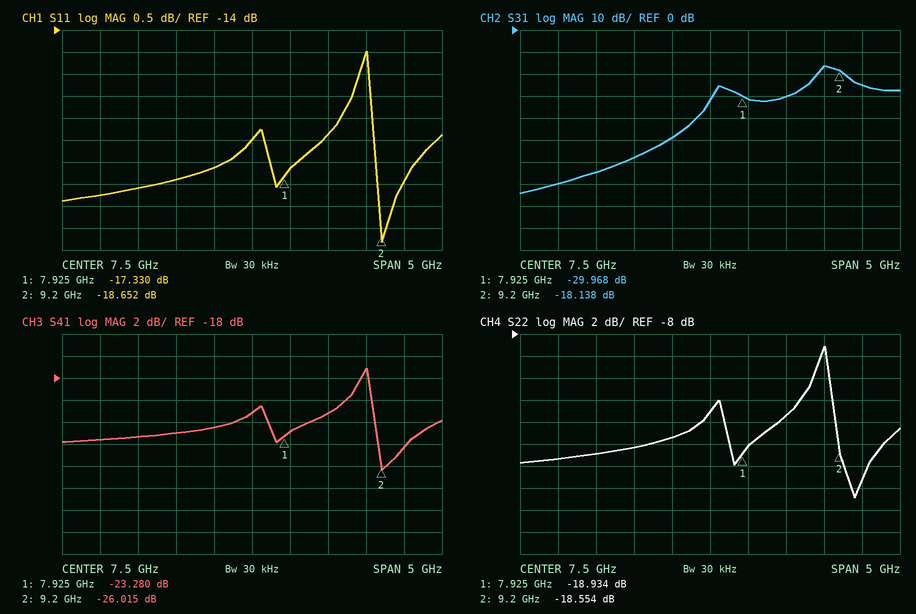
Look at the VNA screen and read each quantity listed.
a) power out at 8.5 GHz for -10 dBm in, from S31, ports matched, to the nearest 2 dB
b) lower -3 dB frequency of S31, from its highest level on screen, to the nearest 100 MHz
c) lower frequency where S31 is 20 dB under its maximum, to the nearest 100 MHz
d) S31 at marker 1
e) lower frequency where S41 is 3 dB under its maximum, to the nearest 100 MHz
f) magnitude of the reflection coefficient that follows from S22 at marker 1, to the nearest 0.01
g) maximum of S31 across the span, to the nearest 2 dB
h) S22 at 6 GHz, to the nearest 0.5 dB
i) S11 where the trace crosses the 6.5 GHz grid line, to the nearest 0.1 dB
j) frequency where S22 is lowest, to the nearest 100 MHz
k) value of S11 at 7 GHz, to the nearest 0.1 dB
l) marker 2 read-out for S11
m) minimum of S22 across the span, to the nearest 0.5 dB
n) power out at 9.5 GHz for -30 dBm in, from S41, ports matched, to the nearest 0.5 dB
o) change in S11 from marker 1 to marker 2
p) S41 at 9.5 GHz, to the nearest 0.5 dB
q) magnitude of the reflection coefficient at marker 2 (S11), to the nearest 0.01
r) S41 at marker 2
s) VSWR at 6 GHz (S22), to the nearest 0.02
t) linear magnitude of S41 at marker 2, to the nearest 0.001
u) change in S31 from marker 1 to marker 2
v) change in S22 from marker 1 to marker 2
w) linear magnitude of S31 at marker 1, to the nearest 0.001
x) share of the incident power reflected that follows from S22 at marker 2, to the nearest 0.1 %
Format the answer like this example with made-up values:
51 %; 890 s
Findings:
-40 dBm; 8.9 GHz; 7.4 GHz; -29.968 dB; 8.7 GHz; 0.11; -16 dB; -19.0 dB; -17.4 dB; 9.4 GHz; -17.1 dB; -18.652 dB; -23.0 dB; -54.5 dBm; -1.322 dB; -24.5 dB; 0.12; -26.015 dB; 1.26; 0.050; 11.830 dB; 0.380 dB; 0.032; 1.4 %
